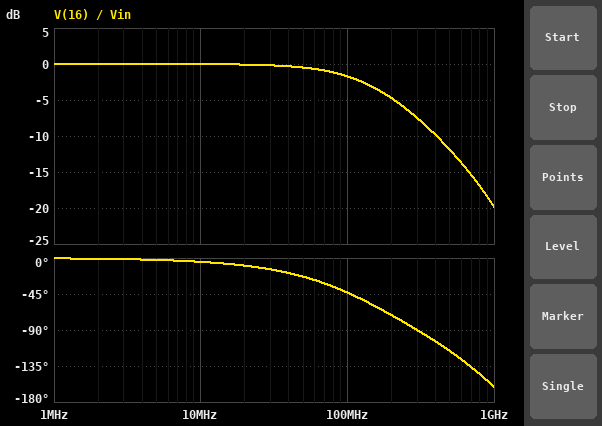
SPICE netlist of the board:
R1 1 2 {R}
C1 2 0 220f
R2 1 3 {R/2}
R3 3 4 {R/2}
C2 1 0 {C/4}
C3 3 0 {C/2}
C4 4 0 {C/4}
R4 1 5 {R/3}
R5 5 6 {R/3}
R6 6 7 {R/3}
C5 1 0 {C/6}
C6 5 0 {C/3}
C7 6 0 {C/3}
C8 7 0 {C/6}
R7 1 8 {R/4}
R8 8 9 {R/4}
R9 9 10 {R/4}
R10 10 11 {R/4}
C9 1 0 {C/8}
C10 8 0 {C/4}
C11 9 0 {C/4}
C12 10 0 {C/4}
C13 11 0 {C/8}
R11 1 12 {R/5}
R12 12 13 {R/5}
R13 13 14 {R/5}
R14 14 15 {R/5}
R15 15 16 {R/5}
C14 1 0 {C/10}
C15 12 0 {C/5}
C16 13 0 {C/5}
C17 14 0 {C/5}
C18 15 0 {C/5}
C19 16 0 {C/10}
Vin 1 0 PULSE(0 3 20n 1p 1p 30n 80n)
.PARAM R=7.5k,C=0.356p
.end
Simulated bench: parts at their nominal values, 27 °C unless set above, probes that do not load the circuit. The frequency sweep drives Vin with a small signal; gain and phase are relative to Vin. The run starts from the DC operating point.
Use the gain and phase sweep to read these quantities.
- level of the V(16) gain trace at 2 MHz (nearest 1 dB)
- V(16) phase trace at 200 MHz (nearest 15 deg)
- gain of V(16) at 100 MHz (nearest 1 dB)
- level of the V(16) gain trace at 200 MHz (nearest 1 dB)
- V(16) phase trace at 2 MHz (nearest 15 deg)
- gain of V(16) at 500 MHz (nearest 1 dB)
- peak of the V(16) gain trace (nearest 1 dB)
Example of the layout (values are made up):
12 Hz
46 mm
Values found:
0 dB
-75 deg
-2 dB
-5 dB
0 deg
-12 dB
0 dB
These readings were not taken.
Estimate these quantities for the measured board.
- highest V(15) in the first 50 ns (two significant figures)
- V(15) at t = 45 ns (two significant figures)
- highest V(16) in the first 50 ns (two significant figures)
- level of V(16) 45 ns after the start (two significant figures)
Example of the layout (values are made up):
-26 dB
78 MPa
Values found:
3.0 V
3.0 V
3.0 V
3.0 V
